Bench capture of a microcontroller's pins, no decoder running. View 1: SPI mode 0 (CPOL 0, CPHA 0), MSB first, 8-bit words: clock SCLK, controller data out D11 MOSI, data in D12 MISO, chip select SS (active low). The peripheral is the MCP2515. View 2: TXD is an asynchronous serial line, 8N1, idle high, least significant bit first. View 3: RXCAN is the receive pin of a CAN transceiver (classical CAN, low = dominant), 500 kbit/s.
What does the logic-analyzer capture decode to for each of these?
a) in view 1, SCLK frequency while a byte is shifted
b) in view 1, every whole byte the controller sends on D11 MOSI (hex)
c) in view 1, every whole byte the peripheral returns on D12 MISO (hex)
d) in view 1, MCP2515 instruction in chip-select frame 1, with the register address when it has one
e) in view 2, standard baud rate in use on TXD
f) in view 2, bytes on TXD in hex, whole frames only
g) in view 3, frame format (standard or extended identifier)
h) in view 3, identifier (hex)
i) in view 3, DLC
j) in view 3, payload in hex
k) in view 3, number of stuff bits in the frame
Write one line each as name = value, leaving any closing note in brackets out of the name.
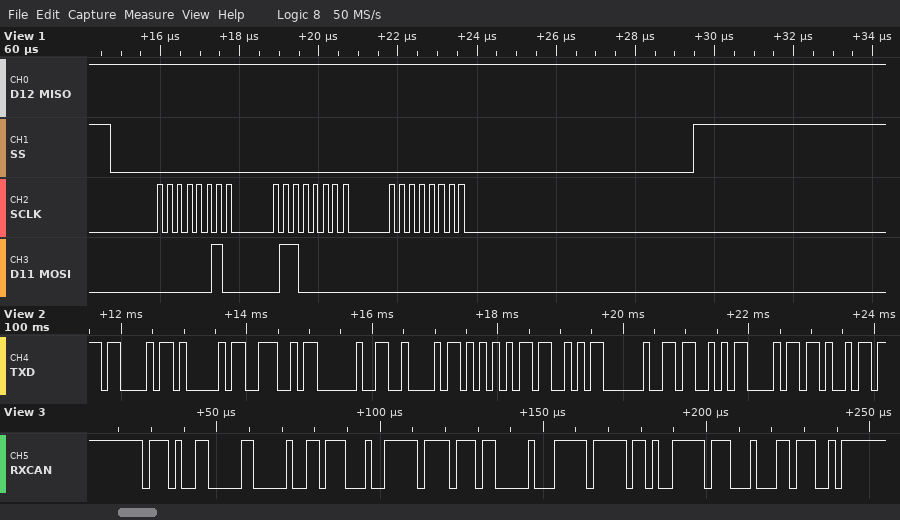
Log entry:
in view 1, SCLK frequency while a byte is shifted = 4 MHz
in view 1, every whole byte the controller sends on D11 MOSI = 02 60 00
in view 1, every whole byte the peripheral returns on D12 MISO = FF FF FF
in view 1, MCP2515 instruction in chip-select frame 1, with the register address when it has one = WRITE 0x60
in view 2, standard baud rate in use on TXD = 9600 baud
in view 2, bytes on TXD in hex, whole frames only = 43 41 4E 20 42 55 53 20 53 68 69
in view 3, frame format = standard
in view 3, identifier = 0x74C
in view 3, DLC = 8
in view 3, payload in hex = 0D C4 FF BB 00 FF F4 FF
in view 3, number of stuff bits in the frame = 7
